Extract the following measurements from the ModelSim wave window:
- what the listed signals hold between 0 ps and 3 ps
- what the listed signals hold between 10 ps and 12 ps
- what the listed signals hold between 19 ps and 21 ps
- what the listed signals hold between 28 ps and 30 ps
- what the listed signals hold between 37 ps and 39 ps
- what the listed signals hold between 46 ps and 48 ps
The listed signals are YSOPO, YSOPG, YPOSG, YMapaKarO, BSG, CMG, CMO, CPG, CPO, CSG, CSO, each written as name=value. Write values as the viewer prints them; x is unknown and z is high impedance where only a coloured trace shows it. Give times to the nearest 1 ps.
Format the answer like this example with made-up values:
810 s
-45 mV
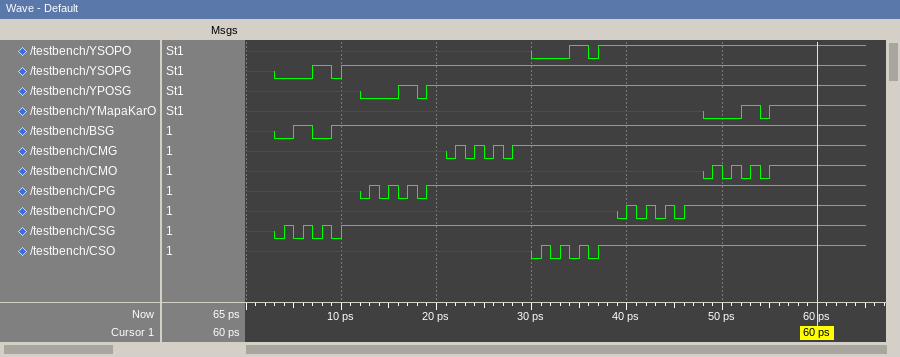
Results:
YSOPO=x, YSOPG=x, YPOSG=x, YMapaKarO=x, BSG=x, CMG=x, CMO=x, CPG=x, CPO=x, CSG=x, CSO=x
YSOPO=x, YSOPG=1, YPOSG=x, YMapaKarO=x, BSG=1, CMG=x, CMO=x, CPG=x, CPO=x, CSG=1, CSO=x
YSOPO=x, YSOPG=1, YPOSG=1, YMapaKarO=x, BSG=1, CMG=x, CMO=x, CPG=1, CPO=x, CSG=1, CSO=x
YSOPO=x, YSOPG=1, YPOSG=1, YMapaKarO=x, BSG=1, CMG=1, CMO=x, CPG=1, CPO=x, CSG=1, CSO=x
YSOPO=1, YSOPG=1, YPOSG=1, YMapaKarO=x, BSG=1, CMG=1, CMO=x, CPG=1, CPO=x, CSG=1, CSO=1
YSOPO=1, YSOPG=1, YPOSG=1, YMapaKarO=x, BSG=1, CMG=1, CMO=x, CPG=1, CPO=1, CSG=1, CSO=1
